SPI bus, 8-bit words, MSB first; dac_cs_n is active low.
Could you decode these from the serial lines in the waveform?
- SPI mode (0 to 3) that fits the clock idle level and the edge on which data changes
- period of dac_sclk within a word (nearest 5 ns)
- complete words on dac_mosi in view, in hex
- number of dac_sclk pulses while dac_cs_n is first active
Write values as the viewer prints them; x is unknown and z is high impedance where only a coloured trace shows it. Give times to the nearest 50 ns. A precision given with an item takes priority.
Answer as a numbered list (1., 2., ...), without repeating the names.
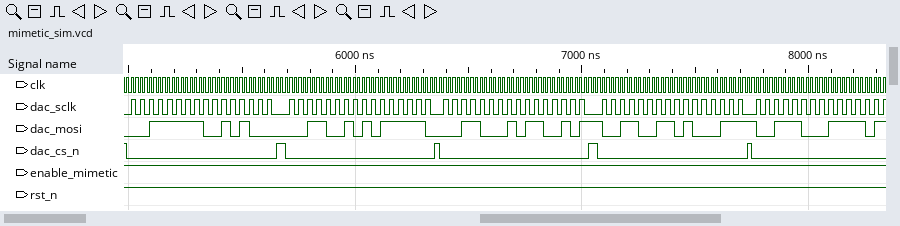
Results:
1. 1
2. 40 ns
3. 3F, 28, 32, BE, 31, 65, 33, 47, 38
4. 16
